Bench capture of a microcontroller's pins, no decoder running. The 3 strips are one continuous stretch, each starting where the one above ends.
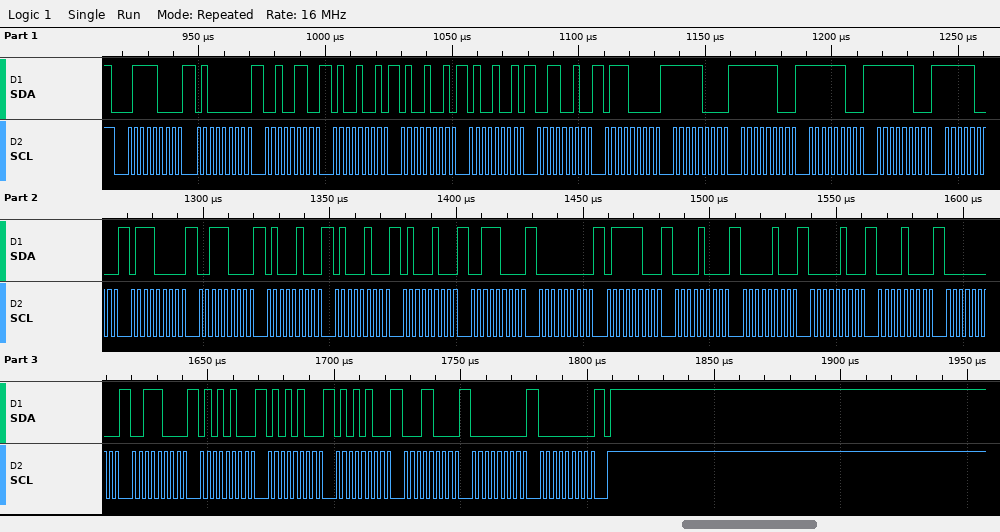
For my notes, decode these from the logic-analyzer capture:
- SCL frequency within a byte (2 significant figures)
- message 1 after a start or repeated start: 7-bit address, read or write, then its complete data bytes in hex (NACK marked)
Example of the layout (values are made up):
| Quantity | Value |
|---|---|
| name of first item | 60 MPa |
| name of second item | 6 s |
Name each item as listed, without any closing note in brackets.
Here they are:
| Quantity | Value |
|---|---|
| SCL frequency within a byte | 400 kHz |
| message 1 after a start or repeated start: 7-bit address, read or write, then its complete data bytes in hex | 0x3C write: 40 26 49 49 49 32 70 F8 FC FC FC F8 70 38 44 44 44 38 00 7C 08 04 04 08 00 38 54 54 54 18 00 00 |
